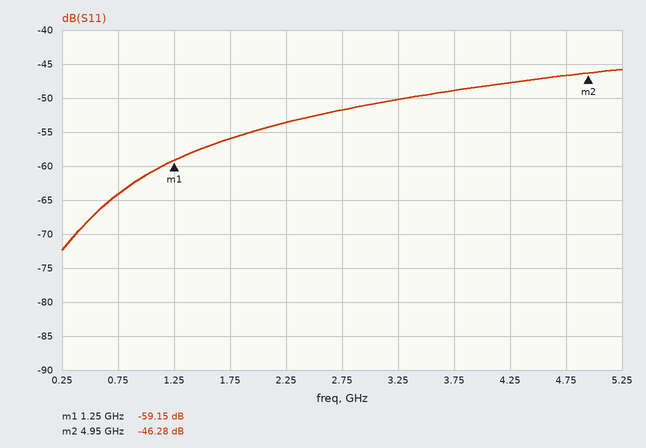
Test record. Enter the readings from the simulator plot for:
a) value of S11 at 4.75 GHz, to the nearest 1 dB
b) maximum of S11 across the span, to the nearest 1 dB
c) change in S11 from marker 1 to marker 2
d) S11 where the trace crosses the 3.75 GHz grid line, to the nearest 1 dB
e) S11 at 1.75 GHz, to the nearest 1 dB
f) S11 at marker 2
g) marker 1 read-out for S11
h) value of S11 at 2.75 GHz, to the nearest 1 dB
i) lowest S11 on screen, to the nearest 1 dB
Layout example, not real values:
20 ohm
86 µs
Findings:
-47 dB
-46 dB
12.87 dB
-49 dB
-56 dB
-46.28 dB
-59.15 dB
-52 dB
-72 dB
